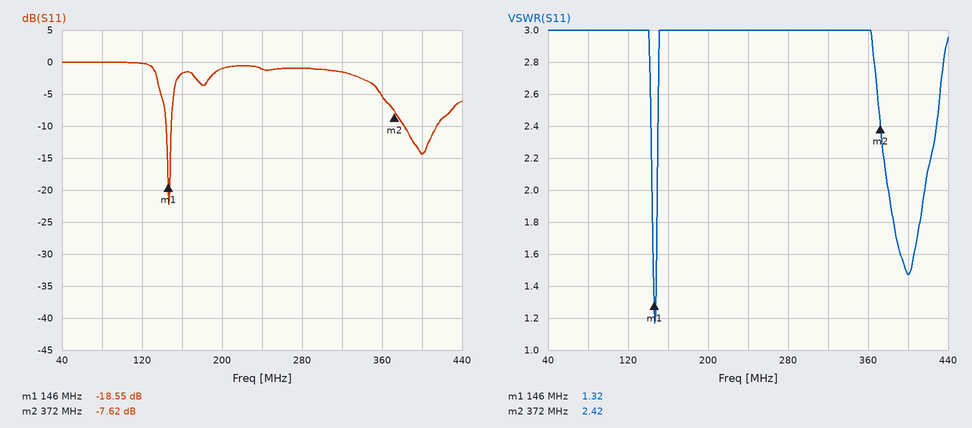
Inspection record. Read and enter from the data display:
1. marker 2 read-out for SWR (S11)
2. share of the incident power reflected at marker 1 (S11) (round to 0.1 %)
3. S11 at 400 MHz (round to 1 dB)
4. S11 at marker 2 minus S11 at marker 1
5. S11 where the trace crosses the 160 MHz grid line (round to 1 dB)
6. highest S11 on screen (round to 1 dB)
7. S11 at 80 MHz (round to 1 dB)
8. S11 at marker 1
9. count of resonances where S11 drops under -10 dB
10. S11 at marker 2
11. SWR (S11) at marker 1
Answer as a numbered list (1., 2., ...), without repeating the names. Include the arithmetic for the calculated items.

1. 2.42
2. 10^(-18.55/10) ≈ 1.4 %
3. -14 dB
4. -7.62 − (-18.55) = 10.93 dB
5. -2 dB
6. 0 dB
7. 0 dB
8. -18.55 dB
9. 2
10. -7.62 dB
11. 1.32
